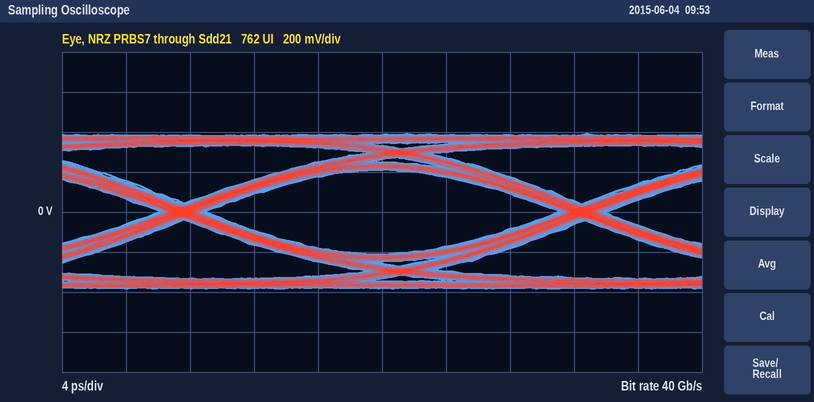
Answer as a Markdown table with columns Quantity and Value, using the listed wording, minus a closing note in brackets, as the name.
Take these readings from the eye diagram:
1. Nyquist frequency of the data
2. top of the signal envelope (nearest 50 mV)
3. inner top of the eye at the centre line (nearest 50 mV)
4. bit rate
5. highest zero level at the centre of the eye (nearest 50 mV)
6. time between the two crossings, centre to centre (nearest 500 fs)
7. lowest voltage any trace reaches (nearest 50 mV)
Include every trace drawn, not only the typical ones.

| Quantity | Value |
|---|---|
| Nyquist frequency of the data | 20 GHz |
| top of the signal envelope | 400 mV |
| inner top of the eye at the centre line | 200 mV |
| bit rate | 40 Gb/s |
| highest zero level at the centre of the eye | -200 mV |
| time between the two crossings, centre to centre | 25.0 ps |
| lowest voltage any trace reaches | -400 mV |
